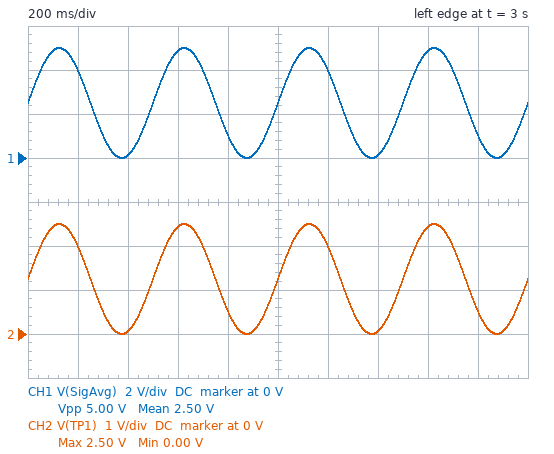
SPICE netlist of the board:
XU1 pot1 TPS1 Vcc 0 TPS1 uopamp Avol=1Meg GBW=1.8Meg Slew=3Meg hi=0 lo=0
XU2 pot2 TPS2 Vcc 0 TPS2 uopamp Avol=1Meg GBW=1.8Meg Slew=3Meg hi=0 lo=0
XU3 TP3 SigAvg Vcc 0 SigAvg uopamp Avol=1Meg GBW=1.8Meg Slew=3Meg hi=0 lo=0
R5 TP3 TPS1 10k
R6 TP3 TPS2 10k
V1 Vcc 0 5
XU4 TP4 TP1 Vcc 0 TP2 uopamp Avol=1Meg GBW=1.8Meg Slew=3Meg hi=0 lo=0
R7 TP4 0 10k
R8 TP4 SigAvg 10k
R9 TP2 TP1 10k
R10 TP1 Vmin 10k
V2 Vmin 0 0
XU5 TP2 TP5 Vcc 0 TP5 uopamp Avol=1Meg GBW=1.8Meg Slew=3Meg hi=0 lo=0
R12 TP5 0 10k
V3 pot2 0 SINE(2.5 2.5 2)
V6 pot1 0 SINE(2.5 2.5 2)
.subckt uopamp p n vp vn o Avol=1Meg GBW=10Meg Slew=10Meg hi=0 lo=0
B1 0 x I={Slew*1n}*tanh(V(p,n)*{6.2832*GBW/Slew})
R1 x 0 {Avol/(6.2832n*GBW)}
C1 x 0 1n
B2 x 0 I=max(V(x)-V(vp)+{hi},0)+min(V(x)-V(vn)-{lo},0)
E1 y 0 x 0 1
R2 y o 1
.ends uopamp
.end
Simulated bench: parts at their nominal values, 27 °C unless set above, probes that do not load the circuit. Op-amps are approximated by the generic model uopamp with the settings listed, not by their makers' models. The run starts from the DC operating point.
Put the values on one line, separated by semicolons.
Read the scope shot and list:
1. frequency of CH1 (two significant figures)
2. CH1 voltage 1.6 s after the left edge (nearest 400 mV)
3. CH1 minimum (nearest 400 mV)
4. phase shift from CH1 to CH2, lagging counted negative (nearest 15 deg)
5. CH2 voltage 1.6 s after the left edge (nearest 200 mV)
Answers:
2.0 Hz; 4.8 V; 0 V; 0 deg; 2.4 V
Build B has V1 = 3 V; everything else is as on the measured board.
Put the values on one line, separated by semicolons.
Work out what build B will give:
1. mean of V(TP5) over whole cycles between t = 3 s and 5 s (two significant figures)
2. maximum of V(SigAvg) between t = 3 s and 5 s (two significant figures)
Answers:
1.9 V; 3.0 V
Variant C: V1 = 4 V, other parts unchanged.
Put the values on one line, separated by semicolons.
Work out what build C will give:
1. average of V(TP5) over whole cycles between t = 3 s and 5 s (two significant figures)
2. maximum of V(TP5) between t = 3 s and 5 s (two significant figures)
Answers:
2.3 V; 4.0 V
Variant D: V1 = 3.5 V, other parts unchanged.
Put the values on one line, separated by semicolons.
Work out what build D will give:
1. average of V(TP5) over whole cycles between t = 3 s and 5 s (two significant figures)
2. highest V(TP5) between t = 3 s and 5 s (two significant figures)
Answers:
2.1 V; 3.5 V
